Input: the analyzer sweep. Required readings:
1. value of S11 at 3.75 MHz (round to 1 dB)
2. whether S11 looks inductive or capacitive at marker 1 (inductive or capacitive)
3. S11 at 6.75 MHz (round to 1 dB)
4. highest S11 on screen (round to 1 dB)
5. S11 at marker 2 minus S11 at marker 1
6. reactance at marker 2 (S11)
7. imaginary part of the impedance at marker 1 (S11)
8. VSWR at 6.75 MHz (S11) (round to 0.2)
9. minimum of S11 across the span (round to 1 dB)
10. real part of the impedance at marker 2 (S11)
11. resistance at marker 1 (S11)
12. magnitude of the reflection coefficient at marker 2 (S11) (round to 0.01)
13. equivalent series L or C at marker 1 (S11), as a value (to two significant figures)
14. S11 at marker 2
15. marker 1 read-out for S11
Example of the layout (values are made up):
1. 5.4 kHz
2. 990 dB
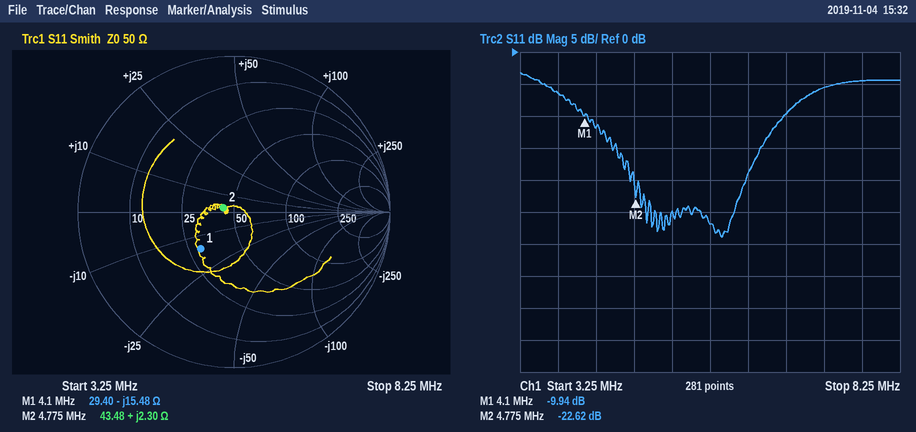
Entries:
1. -6 dB
2. capacitive
3. -10 dB
4. -3 dB
5. -12.68 dB
6. +2.30 Ω
7. -15.48 Ω
8. 2.0
9. -29 dB
10. 43.48 Ω
11. 29.40 Ω
12. 0.07
13. 2.5 nF
14. -22.62 dB
15. -9.94 dB
